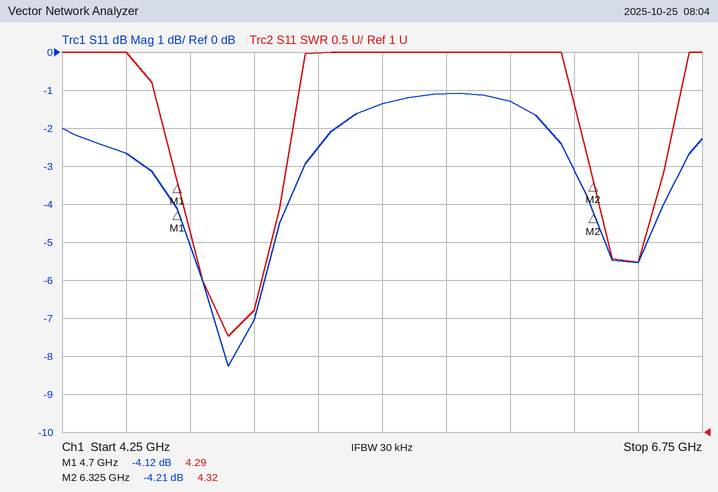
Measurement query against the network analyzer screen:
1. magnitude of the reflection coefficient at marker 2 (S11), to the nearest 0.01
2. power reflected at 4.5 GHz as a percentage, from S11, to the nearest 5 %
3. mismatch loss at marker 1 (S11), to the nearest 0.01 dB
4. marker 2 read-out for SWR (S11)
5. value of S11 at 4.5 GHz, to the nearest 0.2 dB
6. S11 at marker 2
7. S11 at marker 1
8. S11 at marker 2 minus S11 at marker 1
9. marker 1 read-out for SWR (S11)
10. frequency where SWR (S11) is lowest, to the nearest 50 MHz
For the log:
0.62
55 %
2.13 dB
4.32
-2.6 dB
-4.21 dB
-4.12 dB
-0.09 dB
4.29
4.90 GHz
